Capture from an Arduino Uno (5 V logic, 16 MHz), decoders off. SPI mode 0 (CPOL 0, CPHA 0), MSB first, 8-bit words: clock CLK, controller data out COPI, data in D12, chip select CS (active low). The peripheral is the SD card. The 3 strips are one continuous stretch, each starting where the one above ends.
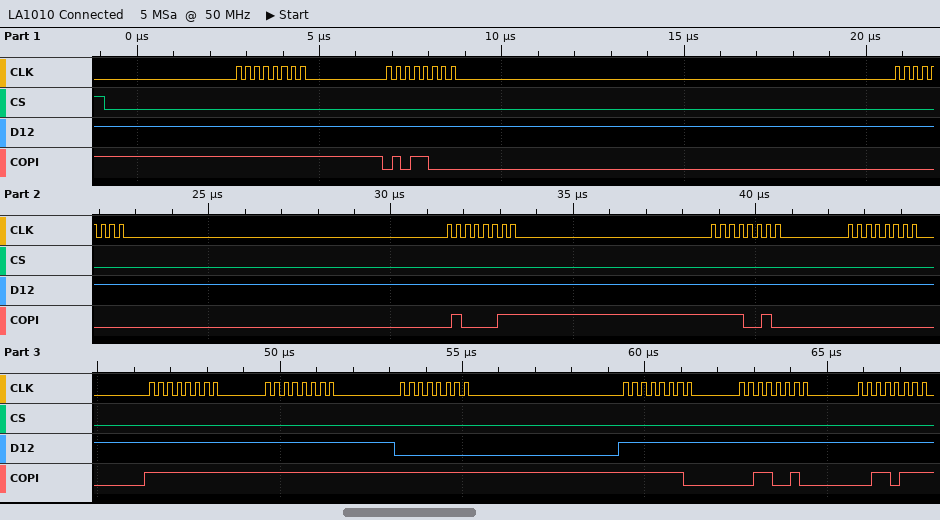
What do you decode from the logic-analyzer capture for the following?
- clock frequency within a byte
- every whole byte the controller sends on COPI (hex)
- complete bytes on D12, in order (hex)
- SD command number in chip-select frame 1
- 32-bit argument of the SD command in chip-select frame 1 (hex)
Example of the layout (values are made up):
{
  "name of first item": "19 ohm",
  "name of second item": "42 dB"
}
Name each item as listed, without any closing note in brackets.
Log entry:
{
  "clock frequency within a byte": "4 MHz",
  "every whole byte the controller sends on COPI": "0xFF 0x58 0x00 0x43 0xF2 0x00 0xFF 0xFF 0xFF 0xFE 0x32 0x37",
  "complete bytes on D12, in order": "0xFF 0xFF 0xFF 0xFF 0xFF 0xFF 0xFF 0xFF 0x00 0xFF 0xFF 0xFF",
  "SD command number in chip-select frame 1": "CMD24",
  "32-bit argument of the SD command in chip-select frame 1": "0x0043F200"
}
